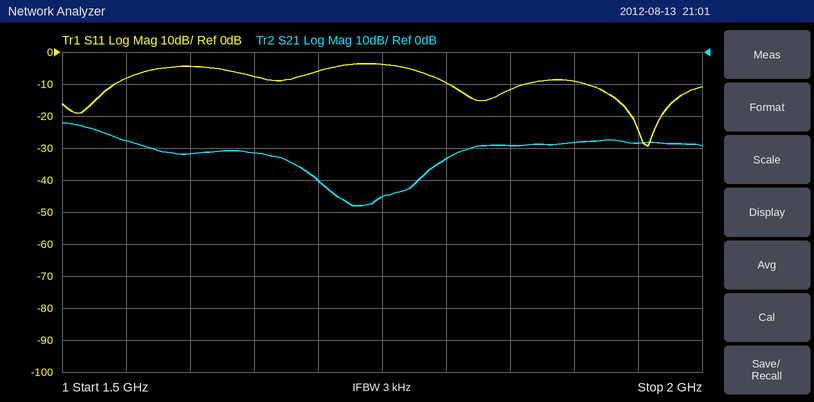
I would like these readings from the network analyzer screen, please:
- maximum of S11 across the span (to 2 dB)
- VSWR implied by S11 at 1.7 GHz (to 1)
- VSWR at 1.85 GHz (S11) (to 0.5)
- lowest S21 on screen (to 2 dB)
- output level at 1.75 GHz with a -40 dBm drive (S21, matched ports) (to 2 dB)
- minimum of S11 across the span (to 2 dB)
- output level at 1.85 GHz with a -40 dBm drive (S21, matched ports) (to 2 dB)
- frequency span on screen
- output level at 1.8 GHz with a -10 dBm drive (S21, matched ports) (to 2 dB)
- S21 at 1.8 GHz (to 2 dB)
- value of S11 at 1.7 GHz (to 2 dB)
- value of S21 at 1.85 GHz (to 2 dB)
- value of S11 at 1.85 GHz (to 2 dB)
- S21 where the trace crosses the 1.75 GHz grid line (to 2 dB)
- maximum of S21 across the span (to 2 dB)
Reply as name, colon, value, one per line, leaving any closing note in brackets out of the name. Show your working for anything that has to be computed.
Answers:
maximum of S11 across the span: -4 dB
VSWR implied by S11 at 1.7 GHz: |Γ| = 10^(-6/20) = 0.5012; VSWR = (1 + 0.5012)/(1 − 0.5012) ≈ 3
VSWR at 1.85 GHz (S11): |Γ| = 10^(-12/20) = 0.2512; VSWR = (1 + 0.2512)/(1 − 0.2512) ≈ 1.67, so 1.5 to the nearest 0.5
lowest S21 on screen: -48 dB
output level at 1.75 GHz with a -40 dBm drive (S21, matched ports): -40 dBm + (-46 dB) = -86 dBm
minimum of S11 across the span: -30 dB
output level at 1.85 GHz with a -40 dBm drive (S21, matched ports): -40 dBm + (-30 dB) = -70 dBm
frequency span on screen: 500 MHz
output level at 1.8 GHz with a -10 dBm drive (S21, matched ports): -10 dBm + (-34 dB) = -44 dBm
S21 at 1.8 GHz: -34 dB
value of S11 at 1.7 GHz: -6 dB
value of S21 at 1.85 GHz: -30 dB
value of S11 at 1.85 GHz: -12 dB
S21 where the trace crosses the 1.75 GHz grid line: -46 dB
maximum of S21 across the span: -22 dB
